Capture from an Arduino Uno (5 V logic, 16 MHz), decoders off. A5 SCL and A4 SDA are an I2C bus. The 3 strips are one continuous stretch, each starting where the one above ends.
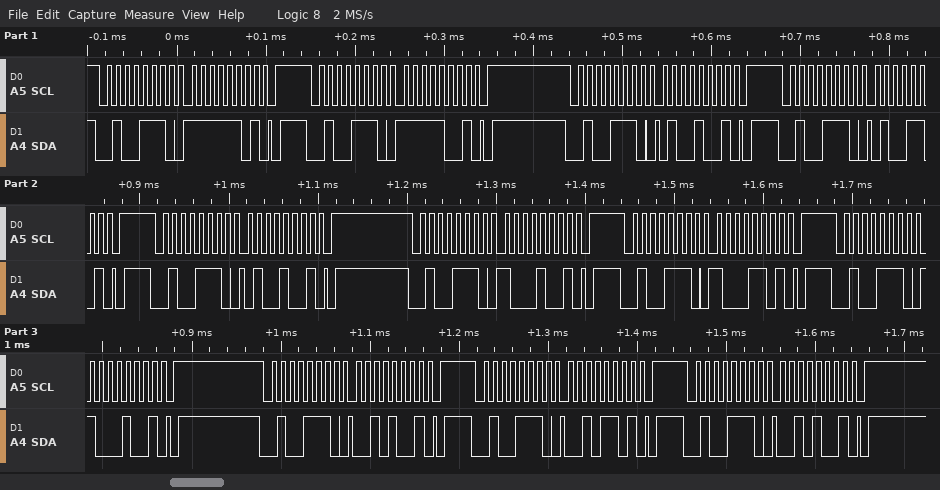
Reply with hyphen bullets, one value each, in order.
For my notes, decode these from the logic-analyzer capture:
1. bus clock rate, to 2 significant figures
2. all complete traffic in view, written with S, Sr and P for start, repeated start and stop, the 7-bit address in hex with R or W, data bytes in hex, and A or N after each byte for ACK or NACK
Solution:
- 100 kHz
- S 27W A FD A P S 27W A F9 A P S 27W A 49 A P S 27W A 4D A P S 27W A 49 A P S 27W A 89 A P S 27W A 8D A P S 27W A 89 A P S 27W A 29 A P S 27W A 2D A P S 27W A 29 A P
